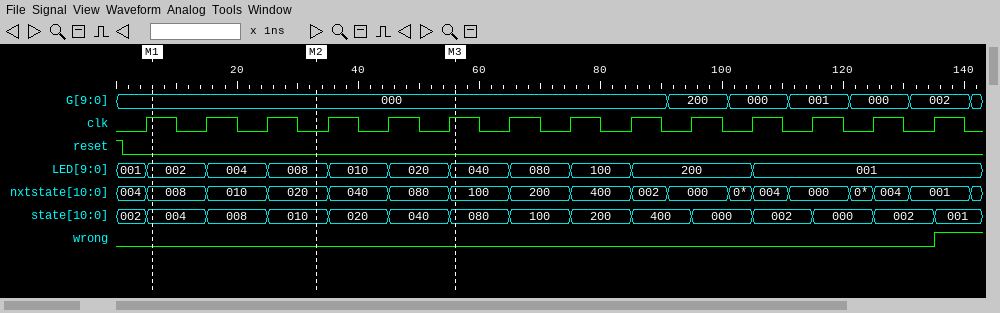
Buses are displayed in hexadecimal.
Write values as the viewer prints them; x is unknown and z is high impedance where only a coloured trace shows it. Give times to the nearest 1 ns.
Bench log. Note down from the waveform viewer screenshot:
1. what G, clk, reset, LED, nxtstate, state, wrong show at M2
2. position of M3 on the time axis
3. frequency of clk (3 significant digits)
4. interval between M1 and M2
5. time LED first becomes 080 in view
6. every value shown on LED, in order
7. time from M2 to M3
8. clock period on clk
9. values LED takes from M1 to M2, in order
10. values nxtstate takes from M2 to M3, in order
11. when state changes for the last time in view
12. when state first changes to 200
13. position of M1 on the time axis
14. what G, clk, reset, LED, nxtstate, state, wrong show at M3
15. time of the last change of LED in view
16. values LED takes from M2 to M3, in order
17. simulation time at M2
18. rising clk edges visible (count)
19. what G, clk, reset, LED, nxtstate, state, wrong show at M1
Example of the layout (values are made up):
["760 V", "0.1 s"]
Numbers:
["G=000, clk=0, reset=0, LED=008, nxtstate=020, state=010, wrong=0", "56 ns", "100 MHz", "27 ns", "65 ns", "001, 002, 004, 008, 010, 020, 040, 080, 100, 200, 001", "23 ns", "10 ns", "002, 004, 008", "020, 040, 080, 100", "135 ns", "75 ns", "6 ns", "G=000, clk=1, reset=0, LED=040, nxtstate=100, state=080, wrong=0", "105 ns", "008, 010, 020, 040", "33 ns", "14", "G=000, clk=1, reset=0, LED=002, nxtstate=008, state=004, wrong=0"]
